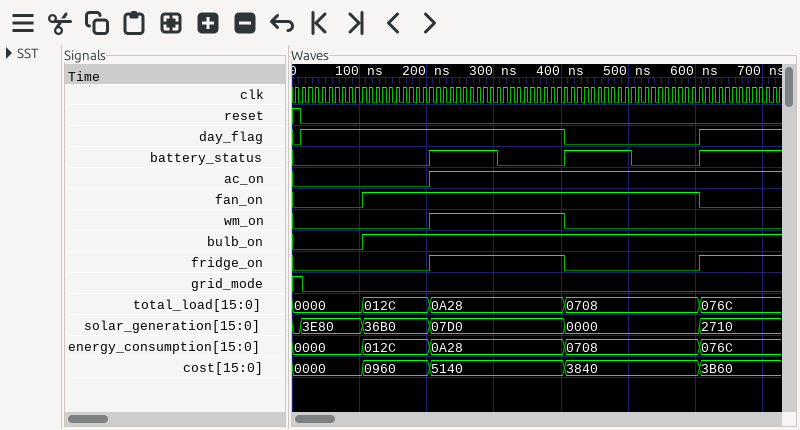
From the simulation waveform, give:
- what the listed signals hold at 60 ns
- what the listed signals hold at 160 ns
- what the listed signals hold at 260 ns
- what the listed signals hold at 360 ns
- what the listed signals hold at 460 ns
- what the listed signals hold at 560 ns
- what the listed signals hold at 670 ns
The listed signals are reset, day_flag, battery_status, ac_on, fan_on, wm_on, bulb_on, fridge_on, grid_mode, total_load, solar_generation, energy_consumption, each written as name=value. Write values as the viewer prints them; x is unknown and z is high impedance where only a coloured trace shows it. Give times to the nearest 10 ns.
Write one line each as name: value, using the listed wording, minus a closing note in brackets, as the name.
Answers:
what the listed signals hold at 60 ns: reset=0, day_flag=1, battery_status=0, ac_on=0, fan_on=0, wm_on=0, bulb_on=0, fridge_on=0, grid_mode=0, total_load=0000, solar_generation=3E80, energy_consumption=0000
what the listed signals hold at 160 ns: reset=0, day_flag=1, battery_status=0, ac_on=0, fan_on=1, wm_on=0, bulb_on=1, fridge_on=0, grid_mode=0, total_load=012C, solar_generation=36B0, energy_consumption=012C
what the listed signals hold at 260 ns: reset=0, day_flag=1, battery_status=1, ac_on=1, fan_on=1, wm_on=1, bulb_on=1, fridge_on=1, grid_mode=0, total_load=0A28, solar_generation=07D0, energy_consumption=0A28
what the listed signals hold at 360 ns: reset=0, day_flag=1, battery_status=0, ac_on=1, fan_on=1, wm_on=1, bulb_on=1, fridge_on=1, grid_mode=0, total_load=0A28, solar_generation=07D0, energy_consumption=0A28
what the listed signals hold at 460 ns: reset=0, day_flag=0, battery_status=1, ac_on=1, fan_on=1, wm_on=0, bulb_on=1, fridge_on=0, grid_mode=0, total_load=0708, solar_generation=0000, energy_consumption=0708
what the listed signals hold at 560 ns: reset=0, day_flag=0, battery_status=0, ac_on=1, fan_on=1, wm_on=0, bulb_on=1, fridge_on=0, grid_mode=0, total_load=0708, solar_generation=0000, energy_consumption=0708
what the listed signals hold at 670 ns: reset=0, day_flag=1, battery_status=1, ac_on=1, fan_on=0, wm_on=0, bulb_on=1, fridge_on=1, grid_mode=0, total_load=076C, solar_generation=2710, energy_consumption=076C
